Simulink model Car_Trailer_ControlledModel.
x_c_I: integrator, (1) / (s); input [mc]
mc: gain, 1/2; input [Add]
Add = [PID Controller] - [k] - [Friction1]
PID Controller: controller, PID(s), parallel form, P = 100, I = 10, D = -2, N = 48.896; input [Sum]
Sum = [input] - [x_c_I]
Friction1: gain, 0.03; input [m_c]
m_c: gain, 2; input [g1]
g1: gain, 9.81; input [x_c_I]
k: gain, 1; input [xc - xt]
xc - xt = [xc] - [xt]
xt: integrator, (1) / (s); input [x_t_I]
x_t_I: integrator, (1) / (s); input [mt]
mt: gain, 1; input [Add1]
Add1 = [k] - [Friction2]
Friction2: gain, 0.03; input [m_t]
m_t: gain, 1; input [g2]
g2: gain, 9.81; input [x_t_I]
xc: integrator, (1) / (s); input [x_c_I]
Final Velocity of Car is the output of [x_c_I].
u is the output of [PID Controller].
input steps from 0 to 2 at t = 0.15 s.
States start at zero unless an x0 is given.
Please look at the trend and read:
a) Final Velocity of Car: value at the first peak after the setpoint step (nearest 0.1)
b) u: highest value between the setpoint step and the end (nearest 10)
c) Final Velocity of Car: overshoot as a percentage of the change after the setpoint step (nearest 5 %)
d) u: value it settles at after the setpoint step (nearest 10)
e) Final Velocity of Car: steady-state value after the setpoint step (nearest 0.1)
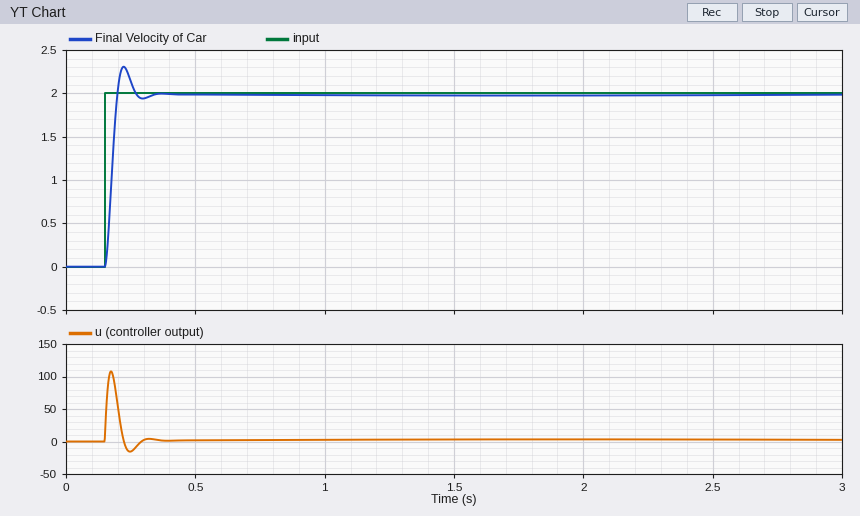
2.3
110
15 %
0
2.0
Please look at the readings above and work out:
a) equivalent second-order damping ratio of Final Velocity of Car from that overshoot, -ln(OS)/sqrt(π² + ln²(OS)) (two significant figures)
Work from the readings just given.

0.52
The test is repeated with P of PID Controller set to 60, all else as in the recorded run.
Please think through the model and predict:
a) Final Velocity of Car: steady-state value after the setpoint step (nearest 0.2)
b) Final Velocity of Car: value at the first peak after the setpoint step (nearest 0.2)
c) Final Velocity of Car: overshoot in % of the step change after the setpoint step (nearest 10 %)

2.0
2.6
30 %
